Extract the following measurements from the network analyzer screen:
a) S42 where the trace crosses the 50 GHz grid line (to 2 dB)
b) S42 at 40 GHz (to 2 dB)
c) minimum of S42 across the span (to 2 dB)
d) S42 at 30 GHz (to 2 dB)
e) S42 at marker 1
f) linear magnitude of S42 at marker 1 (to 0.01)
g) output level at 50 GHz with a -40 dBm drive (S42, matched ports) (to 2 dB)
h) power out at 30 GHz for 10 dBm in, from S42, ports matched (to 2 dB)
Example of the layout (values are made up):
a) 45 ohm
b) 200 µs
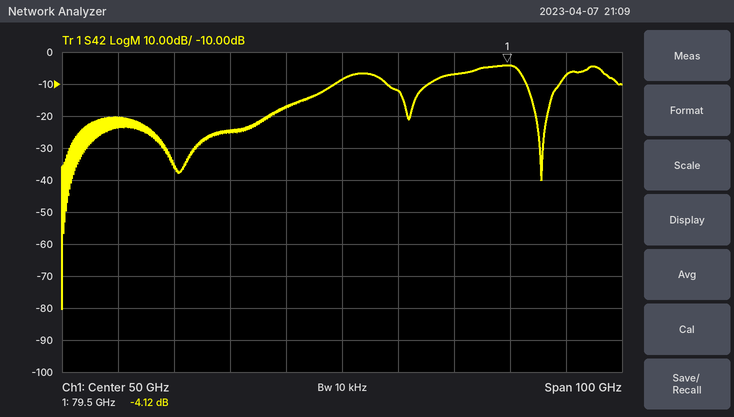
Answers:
a) -8 dB
b) -18 dB
c) -80 dB
d) -24 dB
e) -4.12 dB
f) 0.62
g) -48 dBm
h) -14 dBm
